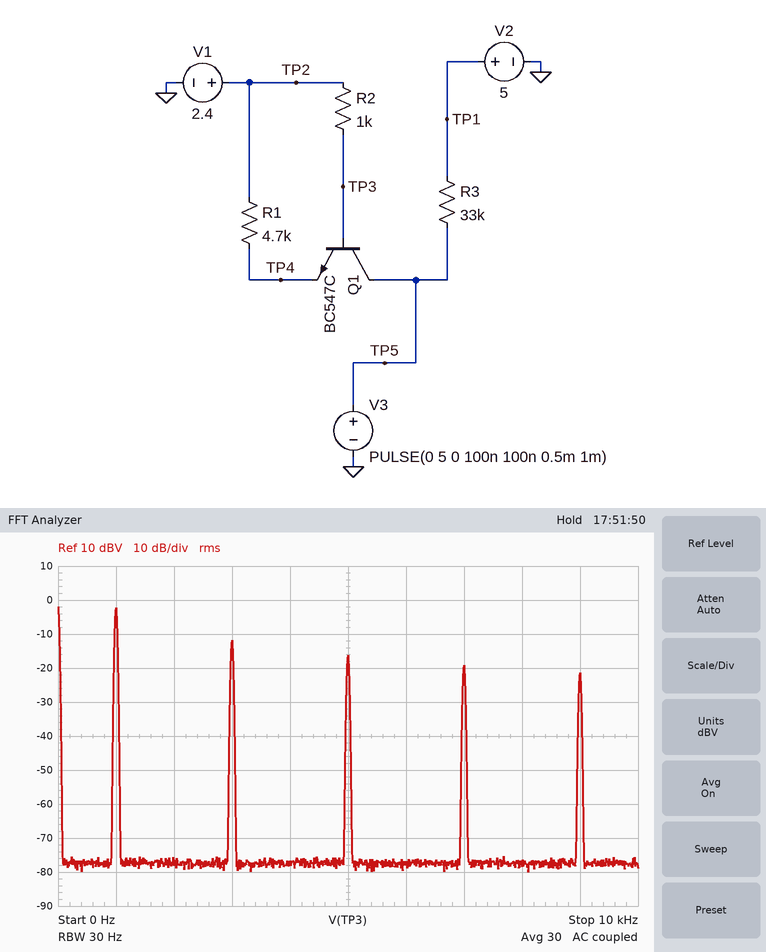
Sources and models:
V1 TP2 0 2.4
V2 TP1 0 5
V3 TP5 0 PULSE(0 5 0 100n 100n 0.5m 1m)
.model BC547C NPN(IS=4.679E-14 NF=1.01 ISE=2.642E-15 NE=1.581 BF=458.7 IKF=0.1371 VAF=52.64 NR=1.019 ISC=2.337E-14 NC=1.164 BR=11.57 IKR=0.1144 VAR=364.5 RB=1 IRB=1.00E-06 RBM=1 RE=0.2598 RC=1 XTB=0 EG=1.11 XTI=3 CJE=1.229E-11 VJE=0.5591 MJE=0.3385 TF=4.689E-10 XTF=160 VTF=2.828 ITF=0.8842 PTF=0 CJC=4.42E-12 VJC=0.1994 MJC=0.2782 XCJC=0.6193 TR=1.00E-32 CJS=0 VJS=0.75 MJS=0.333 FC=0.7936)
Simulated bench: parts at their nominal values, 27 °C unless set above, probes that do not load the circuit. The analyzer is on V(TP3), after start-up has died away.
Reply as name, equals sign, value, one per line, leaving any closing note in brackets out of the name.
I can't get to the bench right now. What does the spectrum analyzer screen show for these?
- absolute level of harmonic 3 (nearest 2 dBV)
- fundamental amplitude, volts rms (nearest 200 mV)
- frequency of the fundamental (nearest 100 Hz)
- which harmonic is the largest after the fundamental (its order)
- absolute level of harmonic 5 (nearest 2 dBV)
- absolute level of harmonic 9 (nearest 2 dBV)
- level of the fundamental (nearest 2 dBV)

absolute level of harmonic 3 = -12 dBV
fundamental amplitude, volts rms = 800 mV
frequency of the fundamental = 1.0 kHz
which harmonic is the largest after the fundamental = 3
absolute level of harmonic 5 = -16 dBV
absolute level of harmonic 9 = -22 dBV
level of the fundamental = -2 dBV
